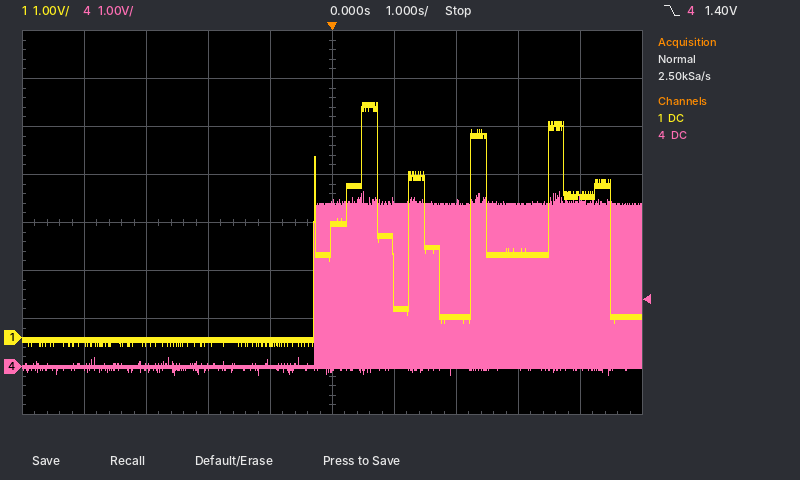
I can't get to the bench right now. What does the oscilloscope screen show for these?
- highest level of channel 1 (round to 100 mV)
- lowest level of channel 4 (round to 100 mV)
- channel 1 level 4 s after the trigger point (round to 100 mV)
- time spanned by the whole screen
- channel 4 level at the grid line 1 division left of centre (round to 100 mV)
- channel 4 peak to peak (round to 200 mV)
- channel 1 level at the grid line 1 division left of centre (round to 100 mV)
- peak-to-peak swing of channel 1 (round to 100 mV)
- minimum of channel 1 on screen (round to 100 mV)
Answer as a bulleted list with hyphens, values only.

- 4.9 V
- -200 mV
- 3.0 V
- 10 s
- 100 mV
- 3.8 V
- -100 mV
- 5.1 V
- -200 mV
